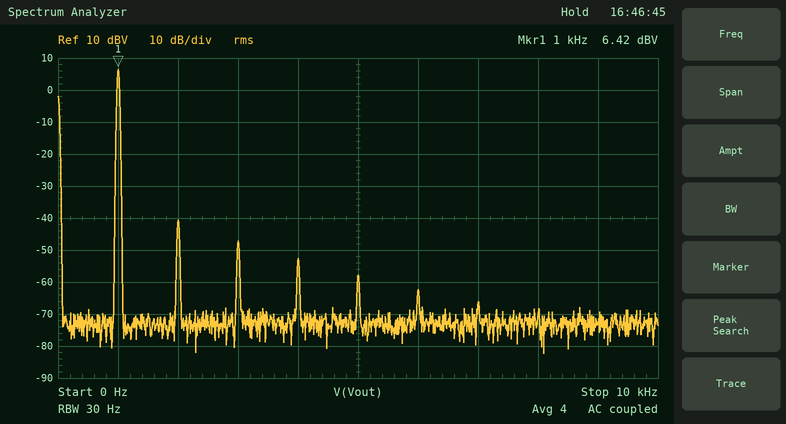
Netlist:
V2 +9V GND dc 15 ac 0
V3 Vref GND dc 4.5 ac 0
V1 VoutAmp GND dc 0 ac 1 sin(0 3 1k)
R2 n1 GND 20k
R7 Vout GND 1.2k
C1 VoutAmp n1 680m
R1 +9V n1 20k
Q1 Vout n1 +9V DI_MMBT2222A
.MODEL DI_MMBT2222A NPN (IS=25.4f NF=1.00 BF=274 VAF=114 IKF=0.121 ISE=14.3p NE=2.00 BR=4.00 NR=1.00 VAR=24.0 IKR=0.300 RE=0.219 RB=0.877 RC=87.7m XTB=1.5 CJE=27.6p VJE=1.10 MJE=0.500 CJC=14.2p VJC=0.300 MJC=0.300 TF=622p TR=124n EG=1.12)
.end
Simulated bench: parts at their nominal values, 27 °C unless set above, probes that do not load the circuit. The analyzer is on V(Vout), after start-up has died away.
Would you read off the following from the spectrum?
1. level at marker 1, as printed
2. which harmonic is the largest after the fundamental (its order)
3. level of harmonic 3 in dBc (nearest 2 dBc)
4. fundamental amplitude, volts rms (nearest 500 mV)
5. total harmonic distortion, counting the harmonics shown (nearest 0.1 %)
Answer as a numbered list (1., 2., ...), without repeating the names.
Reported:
1. 6.42 dBV
2. 2
3. -54 dBc
4. 2.0 V
5. 0.5 %
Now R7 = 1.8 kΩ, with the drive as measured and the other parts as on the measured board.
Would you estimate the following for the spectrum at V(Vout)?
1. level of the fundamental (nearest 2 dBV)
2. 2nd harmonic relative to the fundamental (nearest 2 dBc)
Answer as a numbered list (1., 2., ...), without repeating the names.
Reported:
1. 6 dBV
2. -54 dBc
